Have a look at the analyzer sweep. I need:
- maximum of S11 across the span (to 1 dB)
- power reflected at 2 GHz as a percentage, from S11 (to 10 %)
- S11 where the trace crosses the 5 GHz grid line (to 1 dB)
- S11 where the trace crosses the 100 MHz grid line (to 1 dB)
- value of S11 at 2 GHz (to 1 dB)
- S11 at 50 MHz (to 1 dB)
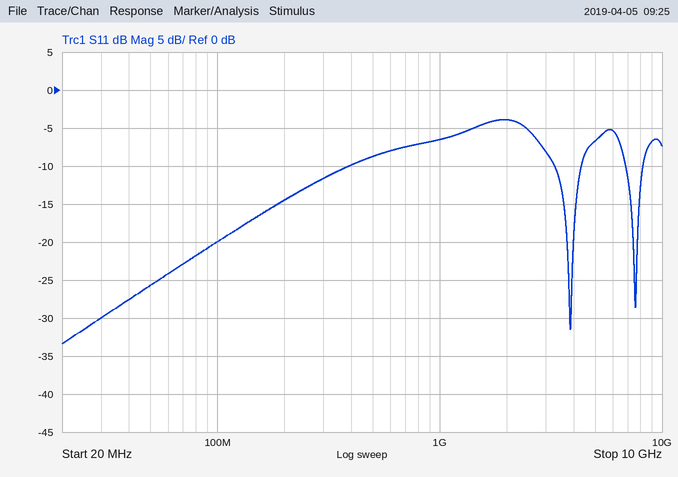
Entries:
-4 dB
40 %
-7 dB
-20 dB
-4 dB
-26 dB
